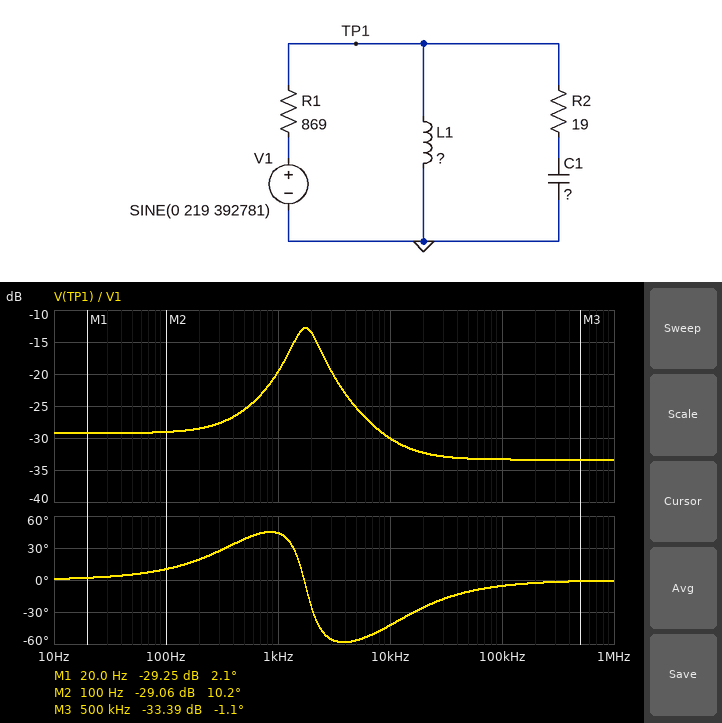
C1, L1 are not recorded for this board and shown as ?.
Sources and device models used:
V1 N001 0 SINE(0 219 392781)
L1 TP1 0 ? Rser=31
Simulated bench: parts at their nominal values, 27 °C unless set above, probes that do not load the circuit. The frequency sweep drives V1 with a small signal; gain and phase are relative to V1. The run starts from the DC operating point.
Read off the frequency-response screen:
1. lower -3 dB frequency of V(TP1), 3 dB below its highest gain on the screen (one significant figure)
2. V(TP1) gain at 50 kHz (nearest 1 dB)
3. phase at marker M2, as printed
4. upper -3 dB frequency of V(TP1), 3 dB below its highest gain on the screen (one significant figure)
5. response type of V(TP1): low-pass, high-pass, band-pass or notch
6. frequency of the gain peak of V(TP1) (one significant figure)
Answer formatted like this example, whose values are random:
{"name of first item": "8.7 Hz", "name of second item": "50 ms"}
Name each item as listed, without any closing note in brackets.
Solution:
{"lower -3 dB frequency of V(TP1), 3 dB below its highest gain on the screen": "1 kHz", "V(TP1) gain at 50 kHz": "-33 dB", "phase at marker M2, as printed": "10.2 deg", "upper -3 dB frequency of V(TP1), 3 dB below its highest gain on the screen": "2 kHz", "response type of V(TP1): low-pass, high-pass, band-pass or notch": "band-pass", "frequency of the gain peak of V(TP1)": "2 kHz"}
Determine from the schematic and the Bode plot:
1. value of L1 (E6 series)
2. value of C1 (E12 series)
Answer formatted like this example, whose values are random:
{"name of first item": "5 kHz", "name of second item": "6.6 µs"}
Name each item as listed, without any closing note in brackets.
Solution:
{"value of L1": "10 mH", "value of C1": "820 nF"}
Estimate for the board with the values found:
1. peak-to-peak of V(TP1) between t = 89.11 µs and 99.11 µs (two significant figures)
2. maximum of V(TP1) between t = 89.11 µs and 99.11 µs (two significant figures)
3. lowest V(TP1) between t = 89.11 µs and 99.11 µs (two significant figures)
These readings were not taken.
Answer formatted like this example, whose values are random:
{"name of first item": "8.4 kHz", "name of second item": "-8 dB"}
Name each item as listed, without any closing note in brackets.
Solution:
{"peak-to-peak of V(TP1) between t = 89.11 µs and 99.11 µs": "9.4 V", "maximum of V(TP1) between t = 89.11 µs and 99.11 µs": "4.7 V", "lowest V(TP1) between t = 89.11 µs and 99.11 µs": "-4.7 V"}
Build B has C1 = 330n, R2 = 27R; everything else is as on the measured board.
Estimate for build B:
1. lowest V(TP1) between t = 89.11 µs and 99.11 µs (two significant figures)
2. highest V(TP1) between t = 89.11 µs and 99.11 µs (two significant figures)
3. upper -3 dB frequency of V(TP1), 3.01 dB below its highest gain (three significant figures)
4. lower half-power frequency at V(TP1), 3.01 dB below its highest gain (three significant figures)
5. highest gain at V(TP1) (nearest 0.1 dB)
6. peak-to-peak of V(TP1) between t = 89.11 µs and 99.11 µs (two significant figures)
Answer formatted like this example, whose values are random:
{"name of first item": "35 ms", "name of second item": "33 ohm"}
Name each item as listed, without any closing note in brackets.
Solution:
{"lowest V(TP1) between t = 89.11 µs and 99.11 µs": "-6.7 V", "highest V(TP1) between t = 89.11 µs and 99.11 µs": "6.6 V", "upper -3 dB frequency of V(TP1), 3.01 dB below its highest gain": "3.60 kHz", "lower half-power frequency at V(TP1), 3.01 dB below its highest gain": "2.14 kHz", "highest gain at V(TP1)": "-8.4 dB", "peak-to-peak of V(TP1) between t = 89.11 µs and 99.11 µs": "13 V"}
